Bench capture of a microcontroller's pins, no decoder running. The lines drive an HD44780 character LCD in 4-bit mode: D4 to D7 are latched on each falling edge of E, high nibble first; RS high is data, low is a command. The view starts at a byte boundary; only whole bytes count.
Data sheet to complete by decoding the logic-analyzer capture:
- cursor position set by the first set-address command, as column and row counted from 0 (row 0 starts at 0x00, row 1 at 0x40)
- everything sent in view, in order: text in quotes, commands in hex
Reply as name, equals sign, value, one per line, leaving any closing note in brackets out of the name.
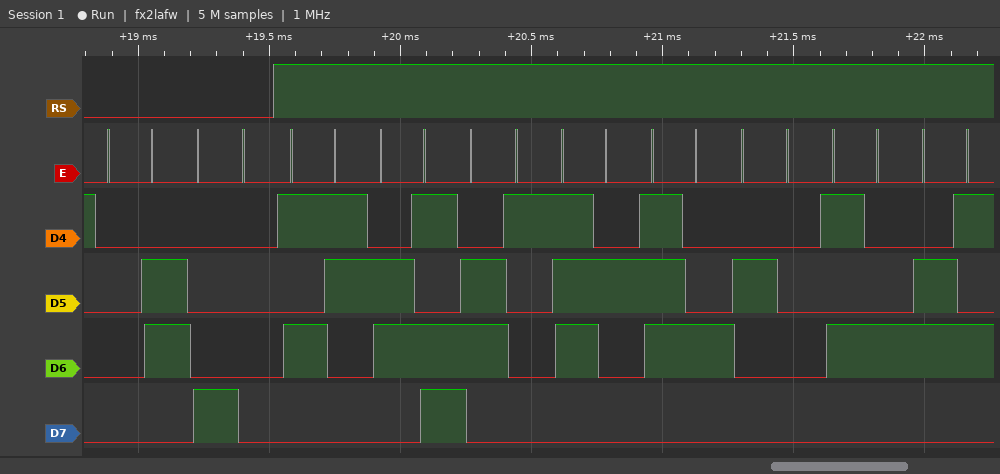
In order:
cursor position set by the first set-address command, as column and row counted from 0 = column 0, row 0
everything sent in view, in order: text in quotes, commands in hex = 0x06 0x80 "Smart Te"
